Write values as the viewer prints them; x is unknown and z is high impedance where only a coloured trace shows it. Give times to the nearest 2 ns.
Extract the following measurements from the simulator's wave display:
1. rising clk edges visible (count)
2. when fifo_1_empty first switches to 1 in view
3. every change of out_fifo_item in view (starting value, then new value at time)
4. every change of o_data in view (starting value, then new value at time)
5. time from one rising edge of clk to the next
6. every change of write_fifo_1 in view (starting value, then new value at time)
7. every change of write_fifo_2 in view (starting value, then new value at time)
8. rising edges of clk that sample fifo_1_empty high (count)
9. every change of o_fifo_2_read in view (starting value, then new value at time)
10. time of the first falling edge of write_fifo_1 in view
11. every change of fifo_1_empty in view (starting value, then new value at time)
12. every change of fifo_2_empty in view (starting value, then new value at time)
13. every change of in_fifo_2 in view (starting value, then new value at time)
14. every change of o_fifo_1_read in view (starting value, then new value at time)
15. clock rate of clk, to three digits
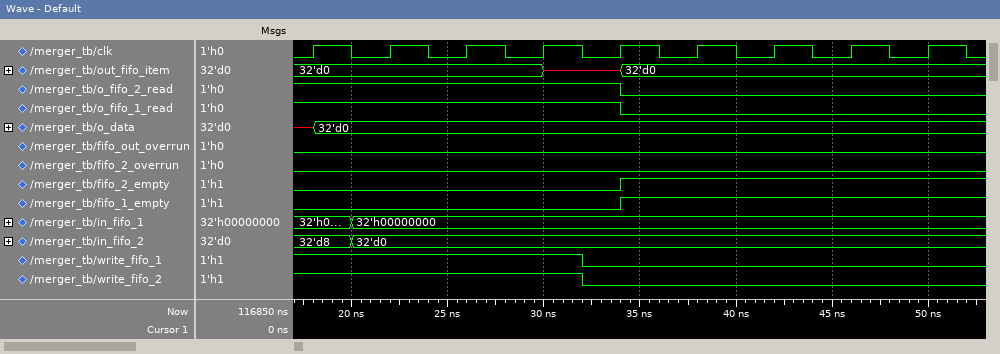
9
34 ns
32'd0, x at 30 ns, 32'd0 at 34 ns
x, 32'd0 at 18 ns
4 ns
1, 0 at 32 ns
1, 0 at 32 ns
4
1, 0 at 34 ns
32 ns
0, 1 at 34 ns
0, 1 at 34 ns
32'd8, 32'd0 at 20 ns
1, 0 at 34 ns
250 MHz
